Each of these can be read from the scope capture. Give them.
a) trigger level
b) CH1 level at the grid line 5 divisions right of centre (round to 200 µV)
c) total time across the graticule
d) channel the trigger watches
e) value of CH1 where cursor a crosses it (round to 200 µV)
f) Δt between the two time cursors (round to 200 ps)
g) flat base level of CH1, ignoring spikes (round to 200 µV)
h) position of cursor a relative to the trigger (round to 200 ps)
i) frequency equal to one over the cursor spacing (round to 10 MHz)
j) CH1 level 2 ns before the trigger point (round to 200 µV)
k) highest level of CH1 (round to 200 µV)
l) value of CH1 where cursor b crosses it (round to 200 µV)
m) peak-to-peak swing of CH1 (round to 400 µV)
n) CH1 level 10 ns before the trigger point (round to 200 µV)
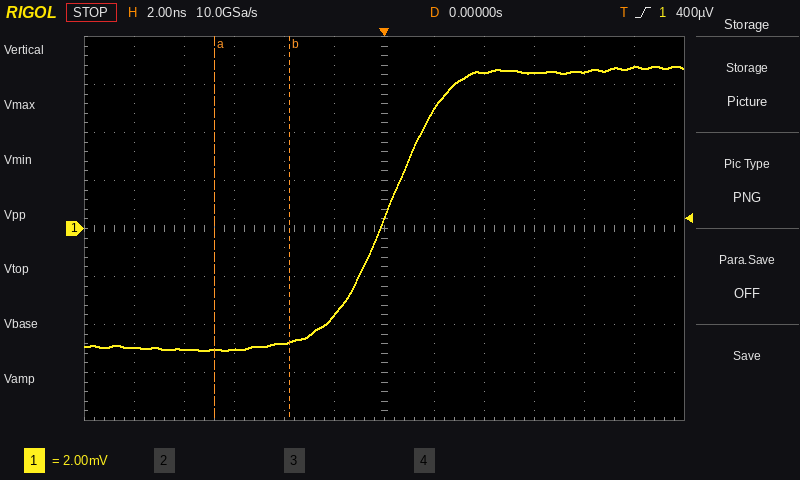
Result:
400 µV
6.8 mV
24 ns
CH1
-5.0 mV
3.0 ns
-5.0 mV
-6.8 ns
330 MHz
-3.6 mV
6.8 mV
-4.8 mV
12.0 mV
-5.0 mV
